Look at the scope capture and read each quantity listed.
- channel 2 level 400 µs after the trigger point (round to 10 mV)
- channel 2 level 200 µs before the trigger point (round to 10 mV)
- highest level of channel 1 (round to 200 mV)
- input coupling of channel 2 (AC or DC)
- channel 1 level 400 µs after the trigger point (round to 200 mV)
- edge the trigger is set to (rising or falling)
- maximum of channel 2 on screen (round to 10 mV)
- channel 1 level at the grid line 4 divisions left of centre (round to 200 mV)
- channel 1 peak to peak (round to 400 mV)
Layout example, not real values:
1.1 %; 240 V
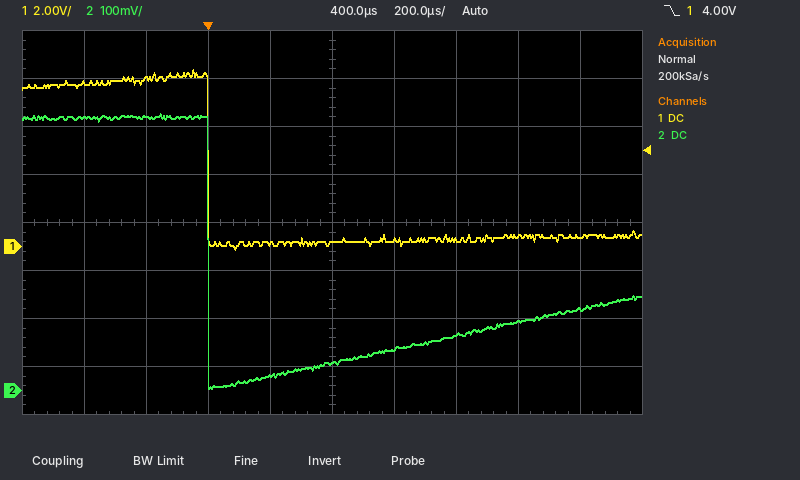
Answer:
60 mV; 570 mV; 7.4 V; DC; 200 mV; falling; 580 mV; 6.8 V; 7.6 V
